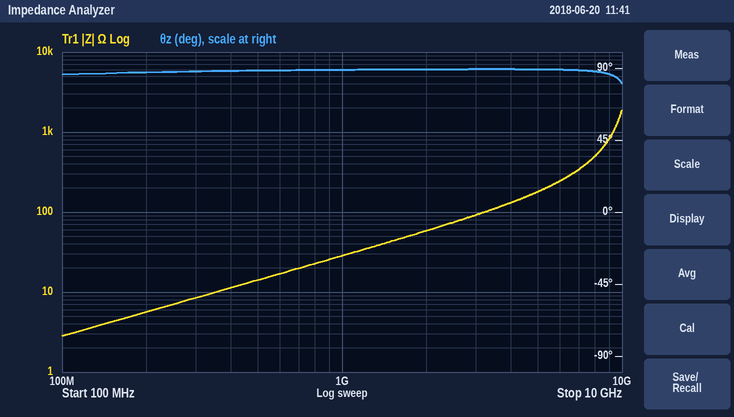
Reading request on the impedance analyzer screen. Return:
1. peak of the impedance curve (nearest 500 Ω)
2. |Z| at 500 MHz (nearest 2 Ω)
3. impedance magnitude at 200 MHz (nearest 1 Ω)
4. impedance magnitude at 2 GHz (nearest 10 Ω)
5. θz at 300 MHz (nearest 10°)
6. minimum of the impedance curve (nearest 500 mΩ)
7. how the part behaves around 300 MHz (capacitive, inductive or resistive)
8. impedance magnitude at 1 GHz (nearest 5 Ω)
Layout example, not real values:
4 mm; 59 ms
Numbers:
2.0 kΩ; 14 Ω; 6 Ω; 60 Ω; 90°; 3.0 Ω; inductive; 30 Ω
